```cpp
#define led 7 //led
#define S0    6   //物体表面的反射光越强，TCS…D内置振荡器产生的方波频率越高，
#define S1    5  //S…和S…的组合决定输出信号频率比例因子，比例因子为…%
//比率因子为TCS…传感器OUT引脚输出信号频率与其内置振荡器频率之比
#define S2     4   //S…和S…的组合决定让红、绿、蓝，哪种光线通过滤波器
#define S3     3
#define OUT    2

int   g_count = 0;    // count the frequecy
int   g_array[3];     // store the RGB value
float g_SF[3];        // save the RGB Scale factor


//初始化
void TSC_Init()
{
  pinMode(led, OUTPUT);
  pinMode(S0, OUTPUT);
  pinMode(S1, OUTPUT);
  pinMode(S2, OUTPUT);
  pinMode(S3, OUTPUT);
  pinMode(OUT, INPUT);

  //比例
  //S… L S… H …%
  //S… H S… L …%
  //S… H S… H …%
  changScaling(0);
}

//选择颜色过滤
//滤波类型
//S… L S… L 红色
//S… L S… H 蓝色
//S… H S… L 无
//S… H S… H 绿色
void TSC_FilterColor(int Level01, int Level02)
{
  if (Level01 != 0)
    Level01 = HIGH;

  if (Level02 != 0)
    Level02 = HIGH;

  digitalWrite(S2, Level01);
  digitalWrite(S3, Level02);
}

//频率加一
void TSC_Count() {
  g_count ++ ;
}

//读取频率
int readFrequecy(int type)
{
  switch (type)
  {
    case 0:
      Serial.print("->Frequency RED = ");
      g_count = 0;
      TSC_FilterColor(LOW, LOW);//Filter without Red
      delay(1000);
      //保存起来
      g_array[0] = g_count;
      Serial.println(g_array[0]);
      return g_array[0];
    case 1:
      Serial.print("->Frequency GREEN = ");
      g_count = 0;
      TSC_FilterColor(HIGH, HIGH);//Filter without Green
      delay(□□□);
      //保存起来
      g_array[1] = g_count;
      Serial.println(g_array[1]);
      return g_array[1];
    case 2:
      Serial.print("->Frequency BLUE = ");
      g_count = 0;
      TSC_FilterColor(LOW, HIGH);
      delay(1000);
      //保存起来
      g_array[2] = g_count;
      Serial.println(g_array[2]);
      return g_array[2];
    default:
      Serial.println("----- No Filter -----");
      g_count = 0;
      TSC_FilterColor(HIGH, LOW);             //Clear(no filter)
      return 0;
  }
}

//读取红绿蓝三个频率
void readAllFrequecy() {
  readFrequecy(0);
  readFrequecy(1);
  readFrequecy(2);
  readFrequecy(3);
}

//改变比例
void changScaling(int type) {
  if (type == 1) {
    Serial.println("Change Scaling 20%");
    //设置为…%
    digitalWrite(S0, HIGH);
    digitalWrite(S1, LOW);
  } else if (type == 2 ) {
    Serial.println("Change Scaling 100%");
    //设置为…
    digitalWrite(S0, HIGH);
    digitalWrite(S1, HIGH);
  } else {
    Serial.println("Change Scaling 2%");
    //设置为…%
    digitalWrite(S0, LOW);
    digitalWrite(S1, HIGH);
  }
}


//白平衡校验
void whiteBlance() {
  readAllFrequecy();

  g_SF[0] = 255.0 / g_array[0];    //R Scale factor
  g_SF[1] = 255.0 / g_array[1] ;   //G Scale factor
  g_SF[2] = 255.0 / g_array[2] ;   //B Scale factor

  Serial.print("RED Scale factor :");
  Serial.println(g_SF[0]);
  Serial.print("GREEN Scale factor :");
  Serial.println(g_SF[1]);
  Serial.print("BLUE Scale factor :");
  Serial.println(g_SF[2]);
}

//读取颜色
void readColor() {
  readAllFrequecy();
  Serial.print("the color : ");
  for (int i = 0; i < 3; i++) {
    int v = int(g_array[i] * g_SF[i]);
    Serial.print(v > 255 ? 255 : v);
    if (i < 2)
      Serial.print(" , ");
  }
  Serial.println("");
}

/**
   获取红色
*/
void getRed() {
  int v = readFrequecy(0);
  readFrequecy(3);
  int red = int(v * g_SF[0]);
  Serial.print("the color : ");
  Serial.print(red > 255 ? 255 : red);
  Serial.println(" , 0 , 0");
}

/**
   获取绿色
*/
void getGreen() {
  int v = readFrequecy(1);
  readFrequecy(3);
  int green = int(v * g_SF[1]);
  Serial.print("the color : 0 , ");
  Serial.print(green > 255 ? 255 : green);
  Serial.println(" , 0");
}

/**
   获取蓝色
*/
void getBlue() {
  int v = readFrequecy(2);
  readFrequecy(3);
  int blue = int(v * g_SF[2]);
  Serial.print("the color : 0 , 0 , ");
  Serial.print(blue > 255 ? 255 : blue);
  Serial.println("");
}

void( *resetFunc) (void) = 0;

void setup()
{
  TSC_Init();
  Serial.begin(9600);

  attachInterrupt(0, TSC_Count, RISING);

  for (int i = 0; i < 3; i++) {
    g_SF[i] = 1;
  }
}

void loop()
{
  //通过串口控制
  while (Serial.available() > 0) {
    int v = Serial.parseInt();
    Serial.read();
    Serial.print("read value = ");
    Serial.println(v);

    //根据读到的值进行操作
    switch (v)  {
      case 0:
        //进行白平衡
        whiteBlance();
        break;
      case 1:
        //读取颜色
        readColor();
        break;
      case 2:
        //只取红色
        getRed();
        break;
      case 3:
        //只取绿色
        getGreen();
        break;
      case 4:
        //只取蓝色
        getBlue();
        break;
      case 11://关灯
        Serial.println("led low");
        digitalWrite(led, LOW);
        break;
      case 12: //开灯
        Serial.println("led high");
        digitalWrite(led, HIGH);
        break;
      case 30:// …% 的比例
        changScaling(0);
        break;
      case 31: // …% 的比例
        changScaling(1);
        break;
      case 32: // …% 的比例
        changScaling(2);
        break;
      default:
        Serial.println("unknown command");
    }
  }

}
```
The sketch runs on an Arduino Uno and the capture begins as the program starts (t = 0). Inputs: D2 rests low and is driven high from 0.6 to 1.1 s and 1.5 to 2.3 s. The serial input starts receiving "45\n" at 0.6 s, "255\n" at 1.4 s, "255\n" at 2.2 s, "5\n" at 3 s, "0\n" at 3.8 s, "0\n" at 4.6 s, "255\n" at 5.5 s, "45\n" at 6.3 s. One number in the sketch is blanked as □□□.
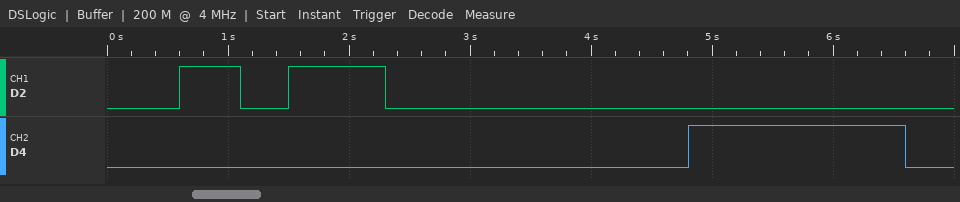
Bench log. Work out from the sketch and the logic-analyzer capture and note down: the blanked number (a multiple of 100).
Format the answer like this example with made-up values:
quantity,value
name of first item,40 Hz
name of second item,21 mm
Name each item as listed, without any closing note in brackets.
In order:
quantity,value
the blanked number,1800
